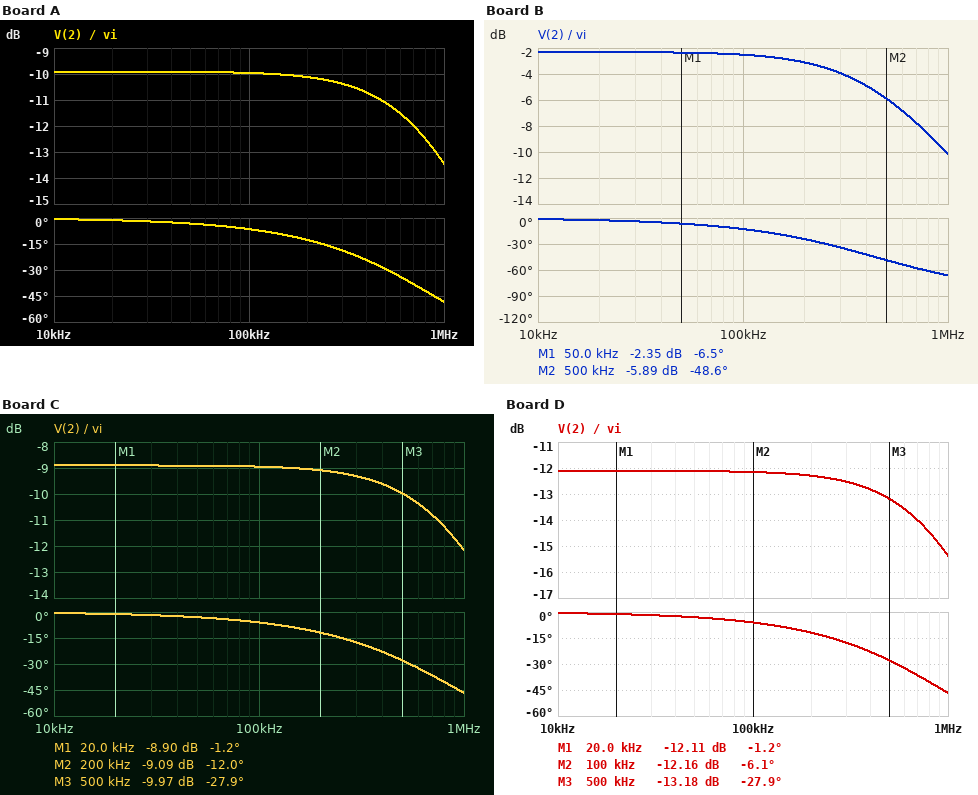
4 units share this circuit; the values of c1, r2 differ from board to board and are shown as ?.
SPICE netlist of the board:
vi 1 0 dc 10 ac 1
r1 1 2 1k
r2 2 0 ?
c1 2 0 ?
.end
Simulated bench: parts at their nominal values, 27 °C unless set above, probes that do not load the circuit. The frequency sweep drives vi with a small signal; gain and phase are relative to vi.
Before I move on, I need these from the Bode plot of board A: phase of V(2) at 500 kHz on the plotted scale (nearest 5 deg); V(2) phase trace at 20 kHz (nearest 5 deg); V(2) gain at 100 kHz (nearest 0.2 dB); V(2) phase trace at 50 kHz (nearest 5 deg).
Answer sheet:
-30 deg
0 deg
-10.0 dB
-5 deg
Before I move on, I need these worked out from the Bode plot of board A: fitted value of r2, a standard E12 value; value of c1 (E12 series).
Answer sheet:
470 Ω
560 pF
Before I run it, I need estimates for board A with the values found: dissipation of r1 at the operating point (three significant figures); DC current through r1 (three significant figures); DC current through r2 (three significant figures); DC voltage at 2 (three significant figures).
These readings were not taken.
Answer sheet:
46.3 mW
6.80 mA
6.80 mA
3.20 V
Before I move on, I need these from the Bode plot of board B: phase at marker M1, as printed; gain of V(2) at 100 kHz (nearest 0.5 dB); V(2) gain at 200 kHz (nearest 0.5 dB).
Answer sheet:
-6.5 deg
-2.5 dB
-3.0 dB
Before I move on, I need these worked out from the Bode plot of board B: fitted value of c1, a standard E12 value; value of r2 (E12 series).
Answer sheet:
470 pF
3.3 kΩ
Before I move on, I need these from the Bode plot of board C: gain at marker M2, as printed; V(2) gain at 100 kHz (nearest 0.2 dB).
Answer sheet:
-9.09 dB
-9.0 dB
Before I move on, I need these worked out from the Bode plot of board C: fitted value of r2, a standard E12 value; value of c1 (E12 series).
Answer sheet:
560 Ω
470 pF
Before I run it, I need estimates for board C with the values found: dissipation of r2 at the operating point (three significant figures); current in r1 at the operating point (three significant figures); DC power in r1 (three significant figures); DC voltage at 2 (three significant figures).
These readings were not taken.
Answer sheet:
23.0 mW
6.41 mA
41.1 mW
3.59 V
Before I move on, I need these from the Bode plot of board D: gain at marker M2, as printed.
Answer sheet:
-12.16 dB
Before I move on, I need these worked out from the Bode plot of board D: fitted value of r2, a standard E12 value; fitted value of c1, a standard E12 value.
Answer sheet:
330 Ω
680 pF
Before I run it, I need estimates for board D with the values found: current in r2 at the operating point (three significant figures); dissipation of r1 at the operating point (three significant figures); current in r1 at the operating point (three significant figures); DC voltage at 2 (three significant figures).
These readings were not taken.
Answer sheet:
7.52 mA
56.5 mW
7.52 mA
2.48 V
